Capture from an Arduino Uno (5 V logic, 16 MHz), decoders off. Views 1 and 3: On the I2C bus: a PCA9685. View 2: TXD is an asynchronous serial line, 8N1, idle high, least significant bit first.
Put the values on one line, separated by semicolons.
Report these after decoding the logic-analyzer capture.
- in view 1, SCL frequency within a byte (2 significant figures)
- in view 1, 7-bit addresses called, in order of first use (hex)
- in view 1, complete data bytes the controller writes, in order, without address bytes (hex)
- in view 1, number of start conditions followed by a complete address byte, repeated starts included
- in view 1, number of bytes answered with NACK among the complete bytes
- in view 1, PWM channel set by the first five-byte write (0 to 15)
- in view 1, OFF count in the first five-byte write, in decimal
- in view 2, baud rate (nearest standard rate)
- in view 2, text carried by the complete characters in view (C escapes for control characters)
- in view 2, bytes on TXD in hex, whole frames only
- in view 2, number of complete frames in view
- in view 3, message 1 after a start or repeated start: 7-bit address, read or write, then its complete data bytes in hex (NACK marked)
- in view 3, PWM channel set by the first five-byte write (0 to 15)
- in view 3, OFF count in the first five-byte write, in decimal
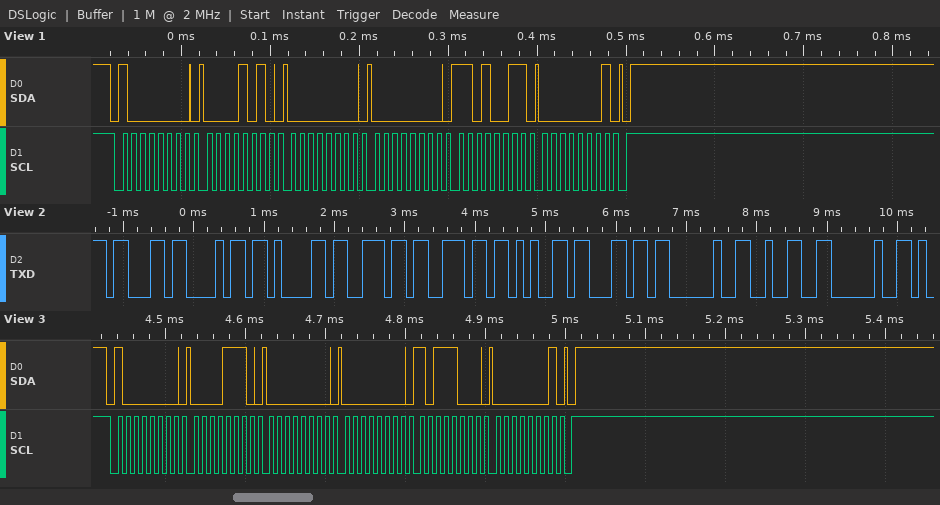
100 kHz; 0x40; 0A 00 00 D3 01; 1; 0; 1; 467; 9600 baud; "channel 2 "; 63 68 61 6E 6E 65 6C 20 32 20; 10; 0x40 write: 0E 00 00 B8 01; 2; 440
